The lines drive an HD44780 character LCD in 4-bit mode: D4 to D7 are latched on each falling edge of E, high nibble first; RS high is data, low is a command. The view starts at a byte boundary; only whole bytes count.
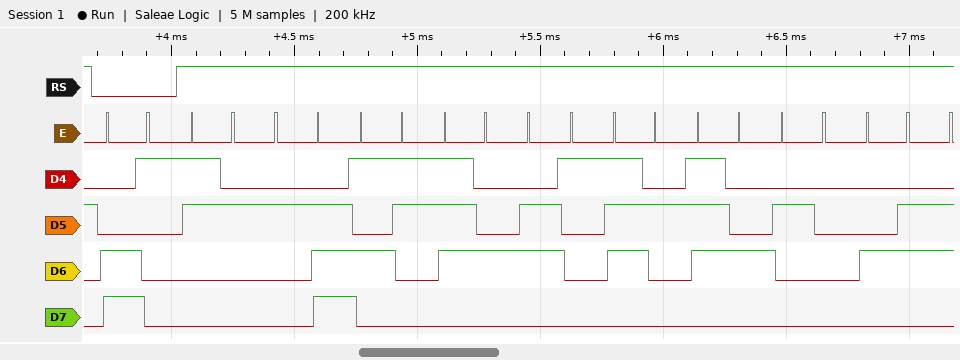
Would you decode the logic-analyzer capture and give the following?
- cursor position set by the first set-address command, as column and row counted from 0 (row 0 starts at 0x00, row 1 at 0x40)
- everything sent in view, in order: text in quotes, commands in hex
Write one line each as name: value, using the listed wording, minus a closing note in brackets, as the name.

cursor position set by the first set-address command, as column and row counted from 0: column 1, row 1
everything sent in view, in order: text in quotes, commands in hex: 0xC1 "2.Start F"
